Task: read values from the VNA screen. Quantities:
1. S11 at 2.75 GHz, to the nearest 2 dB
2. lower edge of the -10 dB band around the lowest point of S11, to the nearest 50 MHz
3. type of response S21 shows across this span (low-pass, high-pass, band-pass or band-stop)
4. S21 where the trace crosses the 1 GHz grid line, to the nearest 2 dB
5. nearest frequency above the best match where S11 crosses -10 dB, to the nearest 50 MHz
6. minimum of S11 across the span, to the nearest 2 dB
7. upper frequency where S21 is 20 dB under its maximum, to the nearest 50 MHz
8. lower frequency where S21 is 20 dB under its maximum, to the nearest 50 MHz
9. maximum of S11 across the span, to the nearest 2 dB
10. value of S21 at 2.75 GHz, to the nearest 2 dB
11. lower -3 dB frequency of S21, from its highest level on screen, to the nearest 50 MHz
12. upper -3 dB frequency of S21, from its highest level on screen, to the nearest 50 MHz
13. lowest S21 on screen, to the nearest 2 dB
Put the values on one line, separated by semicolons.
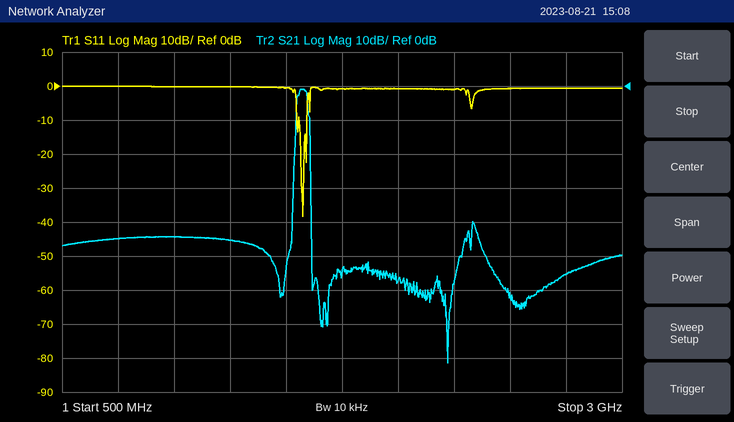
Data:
0 dB; 1.55 GHz; band-pass; -44 dB; 1.60 GHz; -38 dB; 1.60 GHz; 1.55 GHz; 0 dB; -56 dB; 1.55 GHz; 1.60 GHz; -82 dB
